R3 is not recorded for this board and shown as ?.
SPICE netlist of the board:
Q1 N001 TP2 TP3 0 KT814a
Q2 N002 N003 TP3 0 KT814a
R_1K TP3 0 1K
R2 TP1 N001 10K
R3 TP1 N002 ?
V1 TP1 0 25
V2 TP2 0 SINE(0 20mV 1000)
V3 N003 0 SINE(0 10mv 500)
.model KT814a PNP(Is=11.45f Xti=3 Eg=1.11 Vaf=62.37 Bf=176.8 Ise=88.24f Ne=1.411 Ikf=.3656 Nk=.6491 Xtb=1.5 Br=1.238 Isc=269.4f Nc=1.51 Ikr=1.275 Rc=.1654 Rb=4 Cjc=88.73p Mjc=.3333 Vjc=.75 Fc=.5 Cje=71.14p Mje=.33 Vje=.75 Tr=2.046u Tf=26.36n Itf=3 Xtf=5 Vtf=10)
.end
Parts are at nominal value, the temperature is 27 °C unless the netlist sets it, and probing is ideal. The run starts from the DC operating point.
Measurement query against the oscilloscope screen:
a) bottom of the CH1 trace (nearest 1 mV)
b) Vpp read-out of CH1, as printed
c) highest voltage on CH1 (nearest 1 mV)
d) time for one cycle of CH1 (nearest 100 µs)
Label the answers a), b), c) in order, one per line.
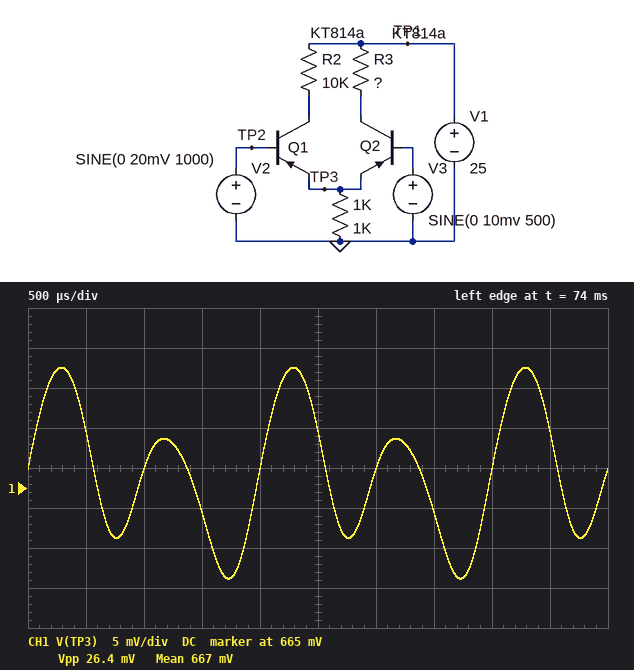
a) 654 mV
b) 26.4 mV
c) 680 mV
d) 1.0 ms
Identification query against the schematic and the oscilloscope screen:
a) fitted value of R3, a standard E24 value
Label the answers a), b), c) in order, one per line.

a) 20 kΩ
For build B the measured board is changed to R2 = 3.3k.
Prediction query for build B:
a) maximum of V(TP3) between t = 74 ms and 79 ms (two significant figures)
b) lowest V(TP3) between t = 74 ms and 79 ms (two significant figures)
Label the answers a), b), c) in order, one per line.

a) 720 mV
b) 690 mV
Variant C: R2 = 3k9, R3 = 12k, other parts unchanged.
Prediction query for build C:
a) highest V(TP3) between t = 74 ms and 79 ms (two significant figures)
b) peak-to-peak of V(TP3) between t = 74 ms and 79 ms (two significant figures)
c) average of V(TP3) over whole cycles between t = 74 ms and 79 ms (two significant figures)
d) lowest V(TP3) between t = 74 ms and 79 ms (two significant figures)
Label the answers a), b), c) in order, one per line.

a) 720 mV
b) 26 mV
c) 700 mV
d) 690 mV
